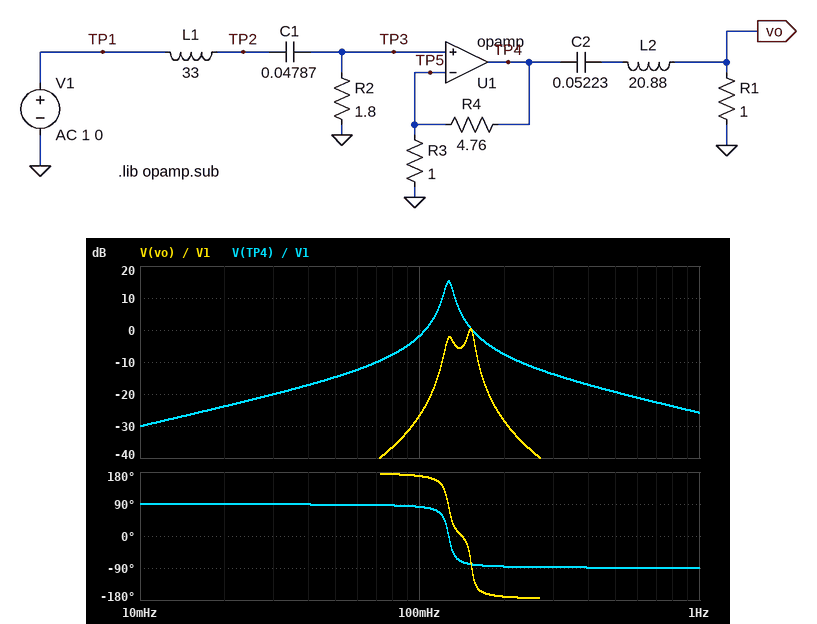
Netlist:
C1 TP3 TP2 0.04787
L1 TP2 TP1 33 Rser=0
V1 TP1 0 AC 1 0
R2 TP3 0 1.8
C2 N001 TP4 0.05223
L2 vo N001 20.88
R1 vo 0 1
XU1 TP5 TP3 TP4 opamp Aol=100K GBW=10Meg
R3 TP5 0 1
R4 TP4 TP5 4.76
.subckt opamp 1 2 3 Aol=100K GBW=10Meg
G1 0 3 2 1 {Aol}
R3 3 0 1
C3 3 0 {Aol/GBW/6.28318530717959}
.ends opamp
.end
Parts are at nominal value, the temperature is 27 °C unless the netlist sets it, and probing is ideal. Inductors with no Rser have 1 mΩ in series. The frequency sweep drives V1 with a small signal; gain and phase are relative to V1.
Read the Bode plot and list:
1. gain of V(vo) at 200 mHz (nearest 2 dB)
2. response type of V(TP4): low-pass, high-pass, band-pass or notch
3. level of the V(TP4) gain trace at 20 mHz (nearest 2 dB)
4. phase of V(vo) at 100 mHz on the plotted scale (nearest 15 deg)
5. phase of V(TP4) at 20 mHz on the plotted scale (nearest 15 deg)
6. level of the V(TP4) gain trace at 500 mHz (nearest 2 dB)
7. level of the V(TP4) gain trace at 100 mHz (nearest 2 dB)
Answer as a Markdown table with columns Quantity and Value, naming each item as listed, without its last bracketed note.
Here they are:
| Quantity | Value |
|---|---|
| gain of V(vo) at 200 mHz | -28 dB |
| response type of V(TP4): low-pass, high-pass, band-pass or notch | band-pass |
| level of the V(TP4) gain trace at 20 mHz | -24 dB |
| phase of V(vo) at 100 mHz on the plotted scale | 165 deg |
| phase of V(TP4) at 20 mHz on the plotted scale | 90 deg |
| level of the V(TP4) gain trace at 500 mHz | -20 dB |
| level of the V(TP4) gain trace at 100 mHz | -2 dB |
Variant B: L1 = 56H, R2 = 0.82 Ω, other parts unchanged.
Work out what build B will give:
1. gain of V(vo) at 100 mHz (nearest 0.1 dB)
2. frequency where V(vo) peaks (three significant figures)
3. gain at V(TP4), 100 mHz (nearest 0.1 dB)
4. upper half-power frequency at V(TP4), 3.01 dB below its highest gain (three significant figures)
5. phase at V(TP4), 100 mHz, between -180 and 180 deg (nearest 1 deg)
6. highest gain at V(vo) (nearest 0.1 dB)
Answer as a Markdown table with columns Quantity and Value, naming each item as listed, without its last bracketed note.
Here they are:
| Quantity | Value |
|---|---|
| gain of V(vo) at 100 mHz | -17.8 dB |
| frequency where V(vo) peaks | 97.2 mHz |
| gain at V(TP4), 100 mHz | 7.0 dB |
| upper half-power frequency at V(TP4), 3.01 dB below its highest gain | 98.4 mHz |
| phase at V(TP4), 100 mHz, between -180 and 180 deg | -67 deg |
| highest gain at V(vo) | -10.2 dB |
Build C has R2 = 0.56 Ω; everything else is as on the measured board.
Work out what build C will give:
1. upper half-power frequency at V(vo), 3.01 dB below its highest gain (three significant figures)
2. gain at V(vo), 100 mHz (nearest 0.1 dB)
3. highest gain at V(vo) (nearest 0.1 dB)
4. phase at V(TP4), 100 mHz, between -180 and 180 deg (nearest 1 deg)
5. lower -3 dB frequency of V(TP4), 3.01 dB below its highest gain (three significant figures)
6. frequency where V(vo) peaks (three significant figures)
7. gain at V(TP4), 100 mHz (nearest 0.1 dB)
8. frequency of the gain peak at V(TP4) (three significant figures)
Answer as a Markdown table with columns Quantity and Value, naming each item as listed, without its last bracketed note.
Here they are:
| Quantity | Value |
|---|---|
| upper half-power frequency at V(vo), 3.01 dB below its highest gain | 128 mHz |
| gain at V(vo), 100 mHz | -36.6 dB |
| highest gain at V(vo) | -2.3 dB |
| phase at V(TP4), 100 mHz, between -180 and 180 deg | 87 deg |
| lower -3 dB frequency of V(TP4), 3.01 dB below its highest gain | 125 mHz |
| frequency where V(vo) peaks | 127 mHz |
| gain at V(TP4), 100 mHz | -11.8 dB |
| frequency of the gain peak at V(TP4) | 127 mHz |
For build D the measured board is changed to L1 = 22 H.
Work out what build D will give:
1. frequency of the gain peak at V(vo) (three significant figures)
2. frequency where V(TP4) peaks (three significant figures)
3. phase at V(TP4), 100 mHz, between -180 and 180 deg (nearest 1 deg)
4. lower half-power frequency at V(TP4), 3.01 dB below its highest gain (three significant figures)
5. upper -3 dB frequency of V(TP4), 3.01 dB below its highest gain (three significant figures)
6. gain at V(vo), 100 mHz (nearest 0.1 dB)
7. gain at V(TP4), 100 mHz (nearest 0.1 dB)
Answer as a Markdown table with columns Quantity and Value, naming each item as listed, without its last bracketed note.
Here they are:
| Quantity | Value |
|---|---|
| frequency of the gain peak at V(vo) | 153 mHz |
| frequency where V(TP4) peaks | 155 mHz |
| phase at V(TP4), 100 mHz, between -180 and 180 deg | 85 deg |
| lower half-power frequency at V(TP4), 3.01 dB below its highest gain | 149 mHz |
| upper -3 dB frequency of V(TP4), 3.01 dB below its highest gain | 162 mHz |
| gain at V(vo), 100 mHz | -30.3 dB |
| gain at V(TP4), 100 mHz | -5.5 dB |
